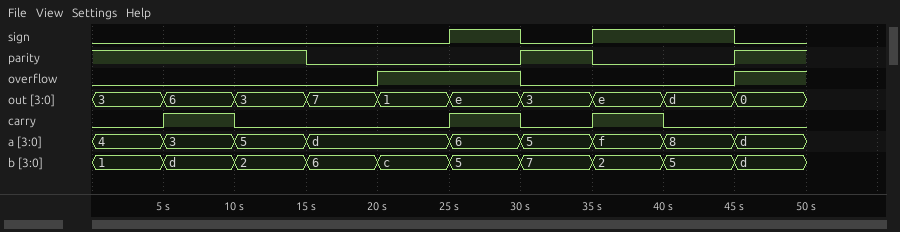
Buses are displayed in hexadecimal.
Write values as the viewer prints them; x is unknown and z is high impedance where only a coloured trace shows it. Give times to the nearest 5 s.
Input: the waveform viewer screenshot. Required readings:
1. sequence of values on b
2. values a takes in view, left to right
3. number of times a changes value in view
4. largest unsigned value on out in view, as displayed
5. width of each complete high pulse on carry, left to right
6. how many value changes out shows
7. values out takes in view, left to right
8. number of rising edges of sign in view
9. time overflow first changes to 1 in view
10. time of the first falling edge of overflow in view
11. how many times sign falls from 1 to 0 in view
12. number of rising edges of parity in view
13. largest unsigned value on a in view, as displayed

1, d, 2, 6, c, 5, 7, 2, 5, d
4, 3, 5, d, 6, 5, f, 8, d
8
e
5 s, 5 s, 5 s
9
3, 6, 3, 7, 1, e, 3, e, d, 0
2
20 s
30 s
2
2
f
